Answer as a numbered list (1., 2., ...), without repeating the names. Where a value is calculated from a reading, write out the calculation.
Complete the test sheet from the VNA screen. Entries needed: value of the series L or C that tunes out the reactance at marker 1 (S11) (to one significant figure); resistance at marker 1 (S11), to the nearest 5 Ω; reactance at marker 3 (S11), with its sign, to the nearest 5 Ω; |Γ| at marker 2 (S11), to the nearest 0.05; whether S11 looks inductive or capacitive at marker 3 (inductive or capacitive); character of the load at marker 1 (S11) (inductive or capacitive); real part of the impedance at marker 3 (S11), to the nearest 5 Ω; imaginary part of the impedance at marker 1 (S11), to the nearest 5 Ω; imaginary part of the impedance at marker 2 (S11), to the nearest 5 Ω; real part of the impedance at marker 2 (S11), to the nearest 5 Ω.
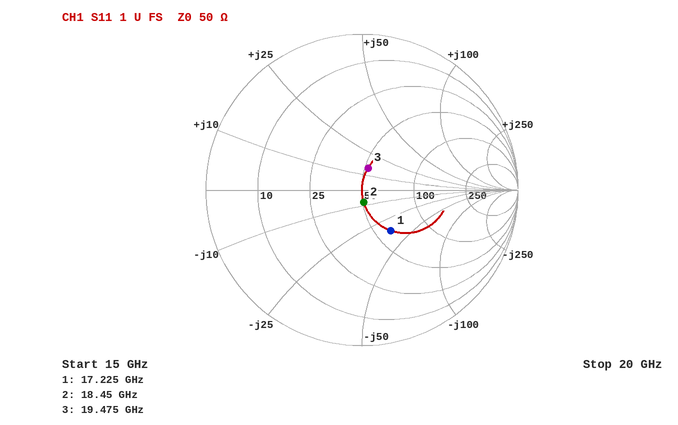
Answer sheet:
1. L = 35 Ω/(2π × 17.225 GHz) ≈ 323 pH, so 300 pH to one significant figure
2. 60 Ω
3. +15 Ω
4. 0.10
5. inductive
6. capacitive
7. 50 Ω
8. -35 Ω
9. -10 Ω
10. 50 Ω
